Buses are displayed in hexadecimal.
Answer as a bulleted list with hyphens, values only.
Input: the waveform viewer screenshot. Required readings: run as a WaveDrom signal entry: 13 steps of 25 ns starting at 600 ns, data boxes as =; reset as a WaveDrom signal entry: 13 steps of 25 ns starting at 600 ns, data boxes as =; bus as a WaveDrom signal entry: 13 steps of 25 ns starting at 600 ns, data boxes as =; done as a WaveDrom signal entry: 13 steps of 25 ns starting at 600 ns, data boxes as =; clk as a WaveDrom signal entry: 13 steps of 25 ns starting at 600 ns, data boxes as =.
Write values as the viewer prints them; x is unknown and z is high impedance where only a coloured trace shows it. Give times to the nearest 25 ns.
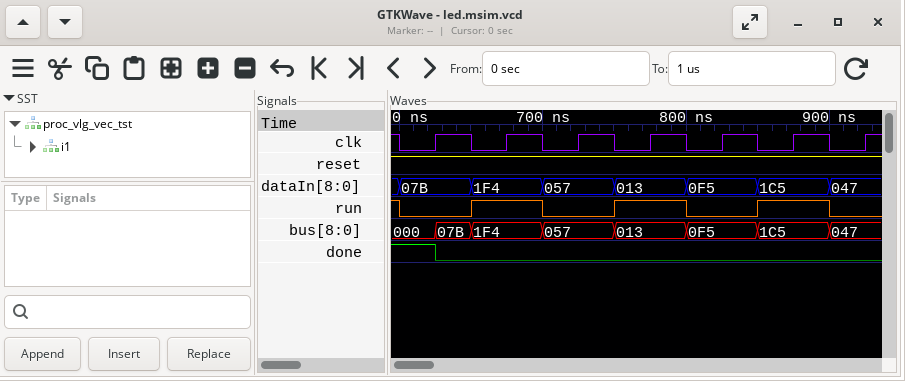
- {name: 'run', wave: '0.1.0.1.0.1.0'}
- {name: 'reset', wave: '1............'}
- {name: 'bus', wave: '===.=.=.=.=.=', data: '000 07B 1F4 057 013 0F5 1C5 047'}
- {name: 'done', wave: '10...........'}
- {name: 'clk', wave: '0101010101010'}
